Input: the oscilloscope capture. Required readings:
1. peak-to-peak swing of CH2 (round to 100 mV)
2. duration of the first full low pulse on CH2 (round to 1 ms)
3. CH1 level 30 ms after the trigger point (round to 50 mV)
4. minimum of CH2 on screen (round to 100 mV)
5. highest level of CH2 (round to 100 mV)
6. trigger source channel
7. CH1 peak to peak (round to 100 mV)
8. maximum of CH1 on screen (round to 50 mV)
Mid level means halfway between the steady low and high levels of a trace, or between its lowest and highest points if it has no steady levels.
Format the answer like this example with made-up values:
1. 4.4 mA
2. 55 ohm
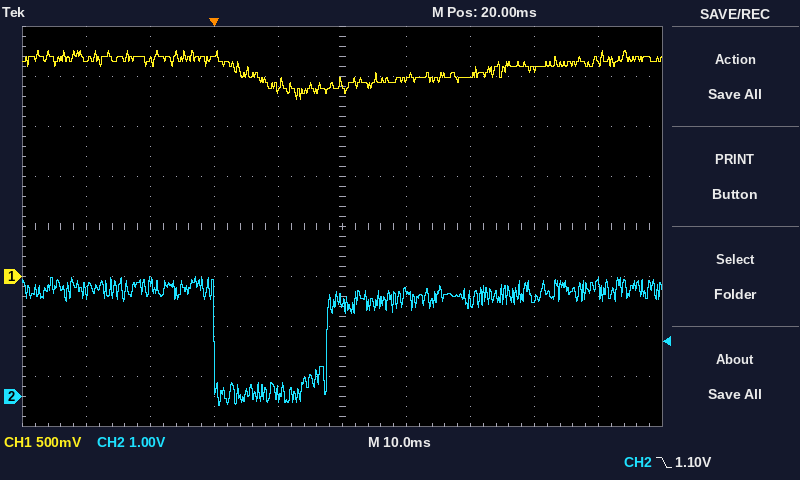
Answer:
1. 2.6 V
2. 18 ms
3. 1.95 V
4. -200 mV
5. 2.4 V
6. CH2
7. 500 mV
8. 2.25 V
